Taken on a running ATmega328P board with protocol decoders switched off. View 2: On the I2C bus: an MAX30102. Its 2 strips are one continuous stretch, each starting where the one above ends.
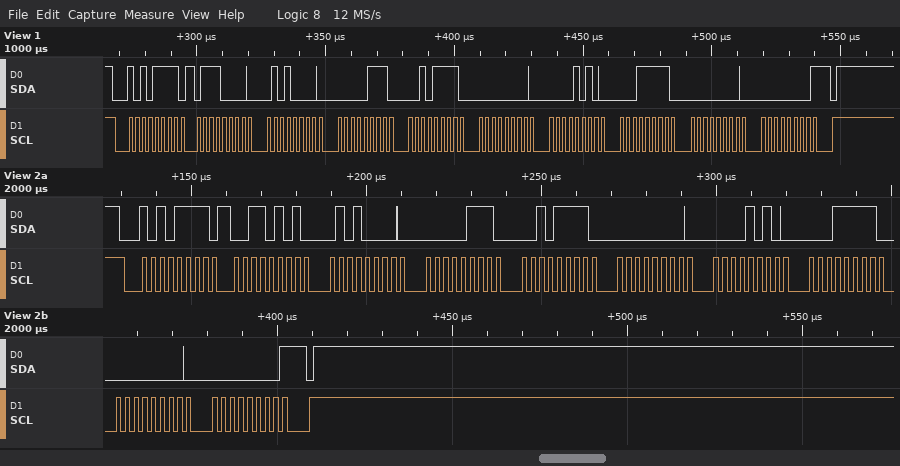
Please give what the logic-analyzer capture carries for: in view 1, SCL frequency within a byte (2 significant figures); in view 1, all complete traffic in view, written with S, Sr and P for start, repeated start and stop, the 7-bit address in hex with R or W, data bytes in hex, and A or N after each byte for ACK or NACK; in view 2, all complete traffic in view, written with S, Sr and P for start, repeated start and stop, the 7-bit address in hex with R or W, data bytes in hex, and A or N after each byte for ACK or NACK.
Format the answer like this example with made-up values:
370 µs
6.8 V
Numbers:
400 kHz
S 57R A 70 A 50 A 07 A 2F A 00 A 0A A 1F A 00 A 00 N P
S 57R A 35 A 50 A 07 A 2F A 00 A 0A A 1F A 00 A 00 N P
